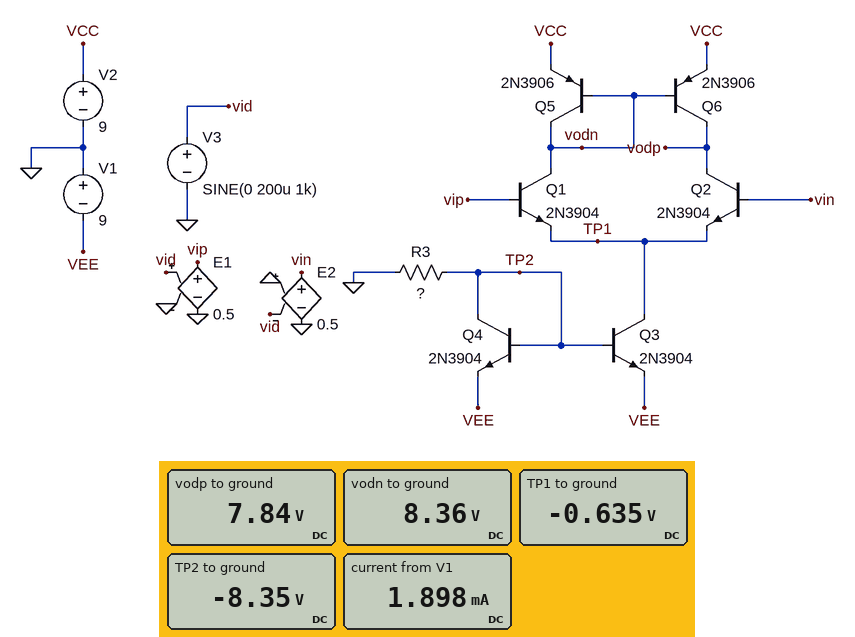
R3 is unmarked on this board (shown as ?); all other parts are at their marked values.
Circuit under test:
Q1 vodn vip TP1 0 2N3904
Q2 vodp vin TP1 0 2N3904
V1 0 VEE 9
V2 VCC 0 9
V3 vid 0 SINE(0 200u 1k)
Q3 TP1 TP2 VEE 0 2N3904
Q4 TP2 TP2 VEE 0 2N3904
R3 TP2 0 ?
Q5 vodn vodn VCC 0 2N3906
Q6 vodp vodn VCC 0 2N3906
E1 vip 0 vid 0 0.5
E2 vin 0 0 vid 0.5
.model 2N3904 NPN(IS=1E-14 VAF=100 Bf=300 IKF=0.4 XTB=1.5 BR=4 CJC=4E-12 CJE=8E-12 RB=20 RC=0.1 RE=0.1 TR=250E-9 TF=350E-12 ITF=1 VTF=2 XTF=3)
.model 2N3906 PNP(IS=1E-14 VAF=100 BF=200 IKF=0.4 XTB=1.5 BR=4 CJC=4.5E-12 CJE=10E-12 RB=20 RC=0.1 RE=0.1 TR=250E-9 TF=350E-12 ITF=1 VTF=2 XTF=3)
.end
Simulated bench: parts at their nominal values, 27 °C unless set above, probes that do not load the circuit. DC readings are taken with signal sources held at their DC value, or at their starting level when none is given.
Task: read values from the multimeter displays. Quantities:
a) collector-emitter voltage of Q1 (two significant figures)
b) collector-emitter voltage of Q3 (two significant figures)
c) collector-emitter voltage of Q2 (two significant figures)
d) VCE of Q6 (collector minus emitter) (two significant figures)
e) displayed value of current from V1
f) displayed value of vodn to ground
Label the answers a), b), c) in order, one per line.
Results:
a) 9.0 V
b) 8.4 V
c) 8.5 V
d) -1.2 V
e) 1.898 mA
f) 8.36 V
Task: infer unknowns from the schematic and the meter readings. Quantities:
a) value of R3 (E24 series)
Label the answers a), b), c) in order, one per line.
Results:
a) 9.1 kΩ
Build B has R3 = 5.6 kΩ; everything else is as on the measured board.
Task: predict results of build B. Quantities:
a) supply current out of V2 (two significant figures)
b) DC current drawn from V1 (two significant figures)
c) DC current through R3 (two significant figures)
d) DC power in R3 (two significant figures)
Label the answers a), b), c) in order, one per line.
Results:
a) 1.6 mA
b) 3.1 mA
c) 1.5 mA
d) 12 mW
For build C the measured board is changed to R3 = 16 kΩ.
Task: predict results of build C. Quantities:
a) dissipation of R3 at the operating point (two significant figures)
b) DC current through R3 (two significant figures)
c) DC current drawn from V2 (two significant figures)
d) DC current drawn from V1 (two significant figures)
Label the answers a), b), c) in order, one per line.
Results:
a) 4.4 mW
b) 520 µA
c) 560 µA
d) 1.1 mA
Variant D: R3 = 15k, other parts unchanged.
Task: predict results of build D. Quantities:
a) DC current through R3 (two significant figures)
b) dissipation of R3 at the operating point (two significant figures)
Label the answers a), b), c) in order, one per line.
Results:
a) 560 µA
b) 4.7 mW
